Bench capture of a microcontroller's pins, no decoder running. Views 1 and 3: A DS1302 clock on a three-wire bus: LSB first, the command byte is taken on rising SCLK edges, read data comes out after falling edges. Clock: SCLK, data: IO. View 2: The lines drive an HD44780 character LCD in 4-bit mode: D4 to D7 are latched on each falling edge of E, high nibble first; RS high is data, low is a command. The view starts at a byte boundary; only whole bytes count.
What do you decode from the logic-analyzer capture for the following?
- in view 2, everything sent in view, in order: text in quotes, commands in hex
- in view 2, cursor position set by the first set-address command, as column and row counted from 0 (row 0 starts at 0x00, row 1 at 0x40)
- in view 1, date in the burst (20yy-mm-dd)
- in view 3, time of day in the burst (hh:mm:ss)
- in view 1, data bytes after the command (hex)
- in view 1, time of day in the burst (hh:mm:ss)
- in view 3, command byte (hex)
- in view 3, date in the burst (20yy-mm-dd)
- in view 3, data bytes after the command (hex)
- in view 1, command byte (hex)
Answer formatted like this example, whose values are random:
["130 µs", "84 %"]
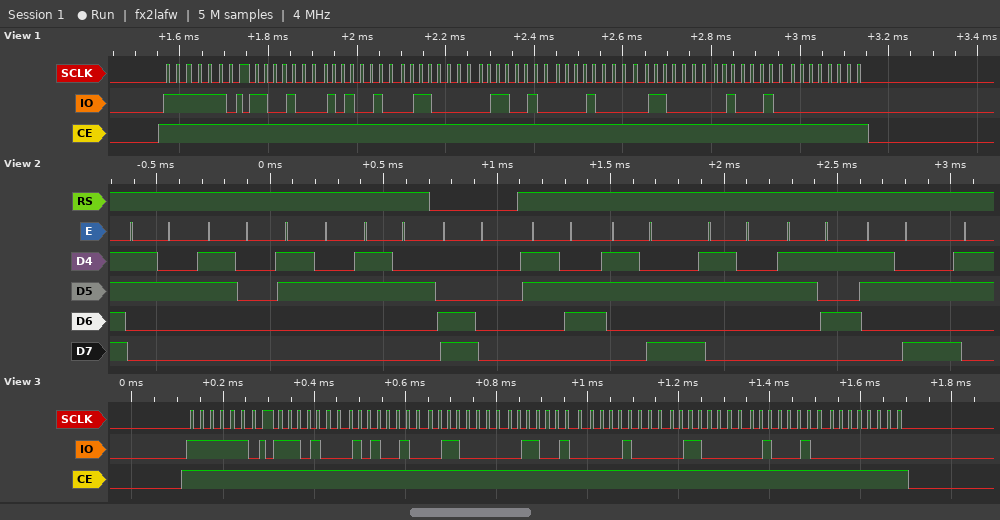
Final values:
["\"2022\" 0xC0 \"6:25:\"", "column 0, row 1", "2022-08-26", "06:25:17", "13 25 06 26 08 06 22 00", "06:25:13", "0xBF", "2022-08-26", "17 25 06 26 08 06 22 00", "0xBF"]
